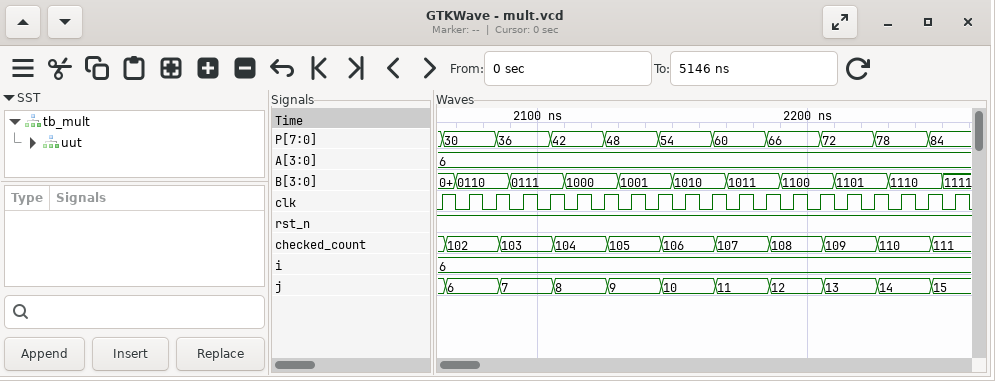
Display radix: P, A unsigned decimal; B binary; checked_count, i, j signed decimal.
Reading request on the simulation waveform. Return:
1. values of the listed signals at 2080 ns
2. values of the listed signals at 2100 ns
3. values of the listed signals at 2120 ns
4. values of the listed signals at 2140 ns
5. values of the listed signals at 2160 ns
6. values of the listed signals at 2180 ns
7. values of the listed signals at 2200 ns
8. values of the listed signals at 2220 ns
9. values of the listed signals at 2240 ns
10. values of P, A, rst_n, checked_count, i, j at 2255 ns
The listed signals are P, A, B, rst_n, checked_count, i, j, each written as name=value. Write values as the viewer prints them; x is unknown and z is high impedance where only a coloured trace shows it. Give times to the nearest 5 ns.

P=30, A=6, B=0110, rst_n=1, checked_count=102, i=6, j=6
P=36, A=6, B=0111, rst_n=1, checked_count=103, i=6, j=7
P=42, A=6, B=1000, rst_n=1, checked_count=104, i=6, j=8
P=48, A=6, B=1001, rst_n=1, checked_count=105, i=6, j=9
P=54, A=6, B=1010, rst_n=1, checked_count=106, i=6, j=10
P=60, A=6, B=1011, rst_n=1, checked_count=107, i=6, j=11
P=66, A=6, B=1100, rst_n=1, checked_count=108, i=6, j=12
P=72, A=6, B=1101, rst_n=1, checked_count=109, i=6, j=13
P=78, A=6, B=1110, rst_n=1, checked_count=110, i=6, j=14
P=84, A=6, rst_n=1, checked_count=111, i=6, j=15
